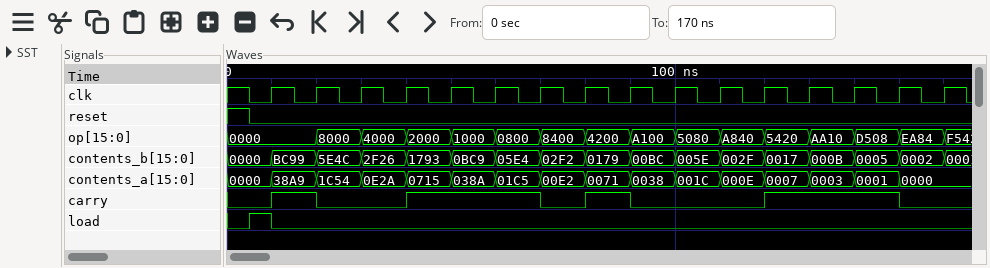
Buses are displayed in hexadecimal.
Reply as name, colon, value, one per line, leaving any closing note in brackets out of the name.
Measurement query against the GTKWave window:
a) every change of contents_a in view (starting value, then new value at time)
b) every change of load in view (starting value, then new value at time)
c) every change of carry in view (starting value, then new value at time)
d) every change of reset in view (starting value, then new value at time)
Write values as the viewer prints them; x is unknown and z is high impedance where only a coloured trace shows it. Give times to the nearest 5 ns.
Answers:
every change of contents_a in view: 0000, 38A9 at 10 ns, 1C54 at 20 ns, 0E2A at 30 ns, 0715 at 40 ns, 038A at 50 ns, 01C5 at 60 ns, 00E2 at 70 ns, 0071 at 80 ns, 0038 at 90 ns, 001C at 100 ns, 000E at 110 ns, 0007 at 120 ns, 0003 at 130 ns, 0001 at 140 ns, 0000 at 150 ns
every change of load in view: 0, 1 at 5 ns, 0 at 10 ns
every change of carry in view: 0, 1 at 10 ns, 0 at 20 ns, 1 at 40 ns, 0 at 70 ns, 1 at 80 ns, 0 at 90 ns, 1 at 120 ns, 0 at 150 ns
every change of reset in view: 1, 0 at 5 ns
